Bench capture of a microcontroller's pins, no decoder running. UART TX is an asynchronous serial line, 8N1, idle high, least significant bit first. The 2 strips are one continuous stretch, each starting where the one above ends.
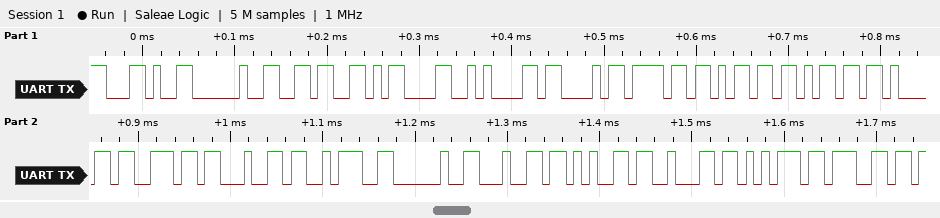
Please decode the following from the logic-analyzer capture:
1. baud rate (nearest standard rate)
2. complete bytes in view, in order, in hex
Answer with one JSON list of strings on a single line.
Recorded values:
["115200 baud", "0x2C 0x20 0x36 0x0D 0x0A 0x43 0x6F 0x6D 0x6D 0x61 0x6E 0x64 0x3A 0x20 0x64 0x65 0x62 0x75 0x67"]
